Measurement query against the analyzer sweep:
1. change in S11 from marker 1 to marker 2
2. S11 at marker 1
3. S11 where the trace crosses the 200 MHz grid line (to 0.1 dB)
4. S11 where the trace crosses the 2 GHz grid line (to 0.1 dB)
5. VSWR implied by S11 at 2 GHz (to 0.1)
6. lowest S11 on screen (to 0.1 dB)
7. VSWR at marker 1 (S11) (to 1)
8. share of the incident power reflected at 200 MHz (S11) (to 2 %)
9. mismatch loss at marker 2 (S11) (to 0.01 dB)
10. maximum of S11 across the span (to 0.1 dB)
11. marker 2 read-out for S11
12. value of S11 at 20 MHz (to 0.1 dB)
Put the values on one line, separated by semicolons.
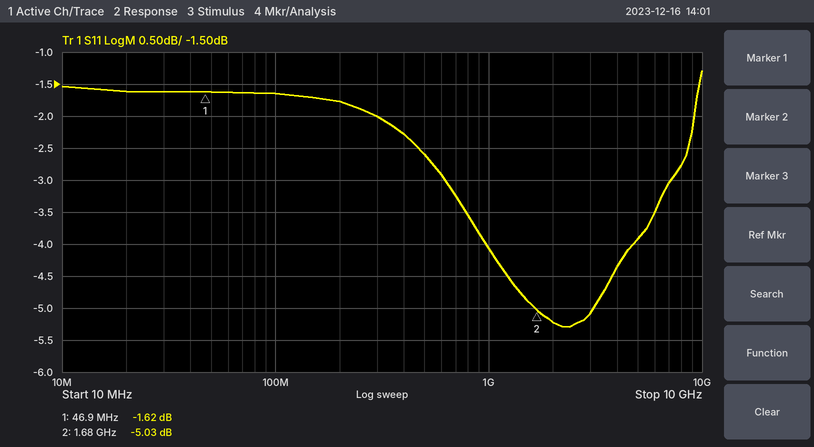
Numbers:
-3.41 dB; -1.62 dB; -1.8 dB; -5.2 dB; 3.4; -5.3 dB; 11; 66 %; 1.64 dB; -1.3 dB; -5.03 dB; -1.6 dB
